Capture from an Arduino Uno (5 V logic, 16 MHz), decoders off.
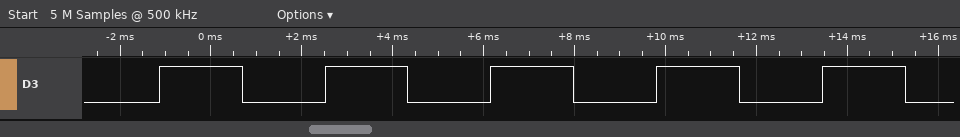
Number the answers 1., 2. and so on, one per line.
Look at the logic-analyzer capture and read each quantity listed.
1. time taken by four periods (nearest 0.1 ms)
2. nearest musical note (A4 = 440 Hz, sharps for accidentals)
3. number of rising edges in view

1. 14.6 ms
2. C#4
3. 5
